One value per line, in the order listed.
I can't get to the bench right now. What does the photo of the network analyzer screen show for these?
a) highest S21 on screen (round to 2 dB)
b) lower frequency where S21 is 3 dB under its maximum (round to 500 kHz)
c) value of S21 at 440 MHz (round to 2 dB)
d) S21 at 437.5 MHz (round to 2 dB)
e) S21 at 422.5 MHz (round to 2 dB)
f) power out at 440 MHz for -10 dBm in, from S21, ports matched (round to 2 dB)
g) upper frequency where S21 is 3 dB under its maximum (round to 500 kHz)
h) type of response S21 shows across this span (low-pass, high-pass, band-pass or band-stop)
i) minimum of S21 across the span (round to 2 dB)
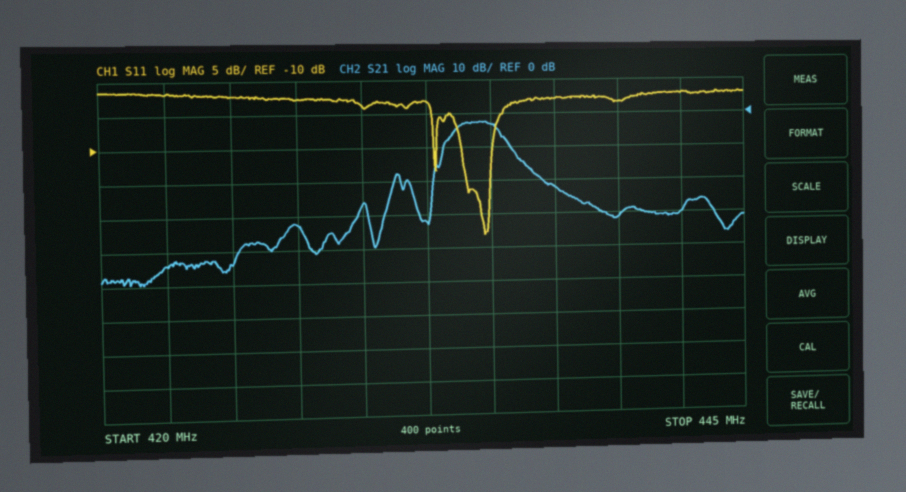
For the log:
-2 dB
433.5 MHz
-32 dB
-22 dB
-44 dB
-42 dBm
435.5 MHz
band-pass
-50 dB
